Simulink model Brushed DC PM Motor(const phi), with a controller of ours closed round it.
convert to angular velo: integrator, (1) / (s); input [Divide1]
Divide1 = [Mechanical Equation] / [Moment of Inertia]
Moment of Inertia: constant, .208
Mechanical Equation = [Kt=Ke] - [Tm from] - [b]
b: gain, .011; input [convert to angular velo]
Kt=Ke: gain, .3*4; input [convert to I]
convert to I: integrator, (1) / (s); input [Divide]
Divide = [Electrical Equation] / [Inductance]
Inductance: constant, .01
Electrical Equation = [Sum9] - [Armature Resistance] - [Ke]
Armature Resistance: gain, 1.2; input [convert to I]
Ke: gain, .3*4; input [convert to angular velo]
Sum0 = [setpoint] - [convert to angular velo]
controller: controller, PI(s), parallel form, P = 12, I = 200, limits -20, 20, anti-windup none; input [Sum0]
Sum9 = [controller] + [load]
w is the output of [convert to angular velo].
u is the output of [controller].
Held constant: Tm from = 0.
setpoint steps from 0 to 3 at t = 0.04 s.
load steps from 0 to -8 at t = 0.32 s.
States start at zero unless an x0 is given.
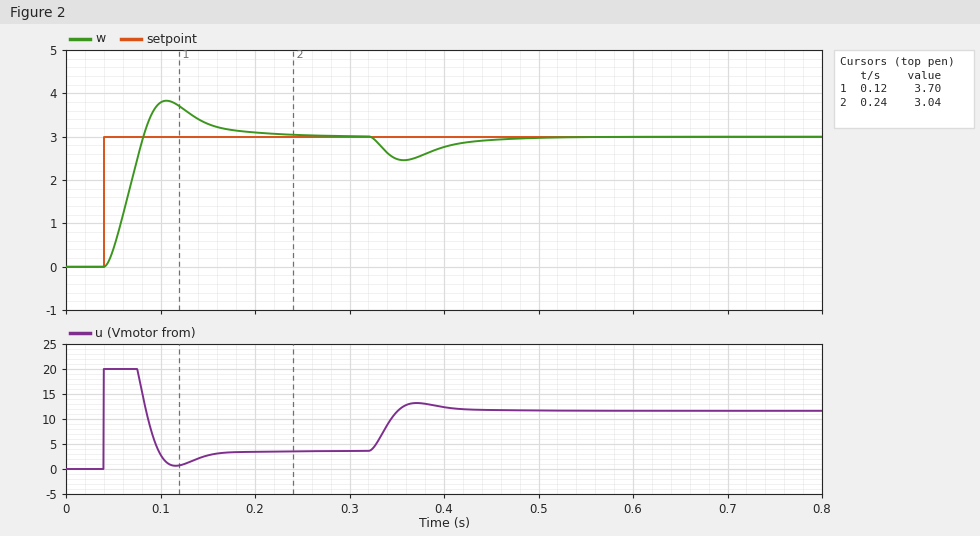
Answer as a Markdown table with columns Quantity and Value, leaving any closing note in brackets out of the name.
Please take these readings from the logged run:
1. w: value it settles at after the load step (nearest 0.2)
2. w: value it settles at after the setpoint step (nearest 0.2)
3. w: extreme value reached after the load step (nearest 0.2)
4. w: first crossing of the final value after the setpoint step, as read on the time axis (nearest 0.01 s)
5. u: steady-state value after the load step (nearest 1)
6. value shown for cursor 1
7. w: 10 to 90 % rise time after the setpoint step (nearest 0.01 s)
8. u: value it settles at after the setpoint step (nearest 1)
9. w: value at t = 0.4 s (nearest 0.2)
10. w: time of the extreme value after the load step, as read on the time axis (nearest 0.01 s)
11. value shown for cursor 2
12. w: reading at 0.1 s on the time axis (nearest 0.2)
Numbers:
| Quantity | Value |
|---|---|
| w: value it settles at after the load step | 3.0 |
| w: value it settles at after the setpoint step | 3.0 |
| w: extreme value reached after the load step | 2.4 |
| w: first crossing of the final value after the setpoint step, as read on the time axis | 0.08 s |
| u: steady-state value after the load step | 12 |
| value shown for cursor 1 | 3.70 |
| w: 10 to 90 % rise time after the setpoint step | 0.03 s |
| u: value it settles at after the setpoint step | 4 |
| w: value at t = 0.4 s | 2.8 |
| w: time of the extreme value after the load step, as read on the time axis | 0.36 s |
| value shown for cursor 2 | 3.04 |
| w: reading at 0.1 s on the time axis | 3.8 |
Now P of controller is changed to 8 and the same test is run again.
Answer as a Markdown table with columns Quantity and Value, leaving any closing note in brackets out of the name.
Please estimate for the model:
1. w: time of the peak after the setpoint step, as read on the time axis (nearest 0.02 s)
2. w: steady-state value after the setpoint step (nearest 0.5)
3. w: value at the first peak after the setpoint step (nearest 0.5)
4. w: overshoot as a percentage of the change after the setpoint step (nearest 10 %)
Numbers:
| Quantity | Value |
|---|---|
| w: time of the peak after the setpoint step, as read on the time axis | 0.12 s |
| w: steady-state value after the setpoint step | 3.0 |
| w: value at the first peak after the setpoint step | 4.0 |
| w: overshoot as a percentage of the change after the setpoint step | 30 % |
